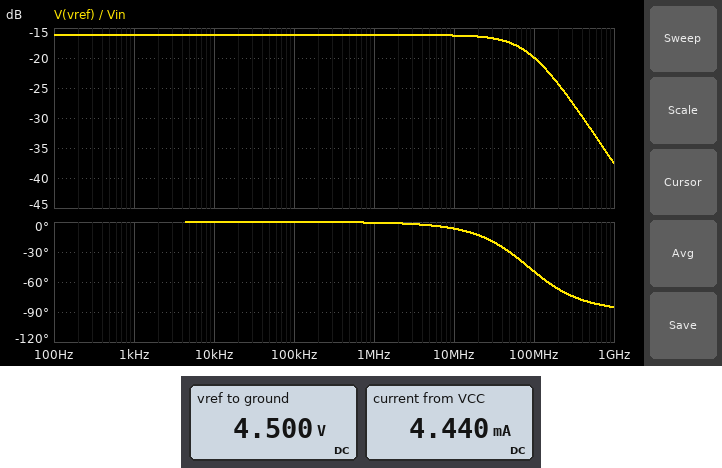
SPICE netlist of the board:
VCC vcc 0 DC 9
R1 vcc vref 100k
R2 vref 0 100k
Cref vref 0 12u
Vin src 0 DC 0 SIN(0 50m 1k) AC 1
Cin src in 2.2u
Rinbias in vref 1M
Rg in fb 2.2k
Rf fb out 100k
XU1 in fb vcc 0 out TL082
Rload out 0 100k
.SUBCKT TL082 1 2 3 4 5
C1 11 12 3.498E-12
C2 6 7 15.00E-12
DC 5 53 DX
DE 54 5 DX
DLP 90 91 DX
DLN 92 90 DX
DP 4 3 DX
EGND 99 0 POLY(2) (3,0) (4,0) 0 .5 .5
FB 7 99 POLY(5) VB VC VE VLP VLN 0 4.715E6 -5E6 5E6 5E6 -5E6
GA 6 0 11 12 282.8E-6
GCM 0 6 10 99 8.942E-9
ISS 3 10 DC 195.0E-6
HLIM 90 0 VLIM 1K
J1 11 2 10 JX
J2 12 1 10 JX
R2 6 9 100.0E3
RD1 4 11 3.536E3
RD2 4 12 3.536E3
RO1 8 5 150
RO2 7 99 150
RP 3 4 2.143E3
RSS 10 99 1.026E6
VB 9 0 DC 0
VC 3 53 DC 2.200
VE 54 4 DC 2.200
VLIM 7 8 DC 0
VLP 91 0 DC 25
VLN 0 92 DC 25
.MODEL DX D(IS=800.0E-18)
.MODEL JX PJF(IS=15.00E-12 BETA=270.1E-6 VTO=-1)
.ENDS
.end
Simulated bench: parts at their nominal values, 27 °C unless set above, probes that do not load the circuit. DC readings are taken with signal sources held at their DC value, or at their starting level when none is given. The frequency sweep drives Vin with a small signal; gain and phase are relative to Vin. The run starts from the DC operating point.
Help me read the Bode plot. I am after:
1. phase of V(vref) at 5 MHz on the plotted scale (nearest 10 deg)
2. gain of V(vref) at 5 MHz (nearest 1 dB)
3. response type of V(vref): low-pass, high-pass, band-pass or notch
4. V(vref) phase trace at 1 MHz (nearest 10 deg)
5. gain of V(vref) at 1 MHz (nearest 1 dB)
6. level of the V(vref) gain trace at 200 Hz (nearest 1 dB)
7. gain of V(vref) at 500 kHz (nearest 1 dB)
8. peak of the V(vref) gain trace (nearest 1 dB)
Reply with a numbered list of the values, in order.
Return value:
1. 0 deg
2. -16 dB
3. low-pass
4. 0 deg
5. -16 dB
6. -16 dB
7. -16 dB
8. -16 dB
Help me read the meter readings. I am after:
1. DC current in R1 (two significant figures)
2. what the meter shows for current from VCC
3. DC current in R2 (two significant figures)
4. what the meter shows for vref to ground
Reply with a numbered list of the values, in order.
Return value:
1. 45 µA
2. 4.440 mA
3. 45 µA
4. 4.500 V
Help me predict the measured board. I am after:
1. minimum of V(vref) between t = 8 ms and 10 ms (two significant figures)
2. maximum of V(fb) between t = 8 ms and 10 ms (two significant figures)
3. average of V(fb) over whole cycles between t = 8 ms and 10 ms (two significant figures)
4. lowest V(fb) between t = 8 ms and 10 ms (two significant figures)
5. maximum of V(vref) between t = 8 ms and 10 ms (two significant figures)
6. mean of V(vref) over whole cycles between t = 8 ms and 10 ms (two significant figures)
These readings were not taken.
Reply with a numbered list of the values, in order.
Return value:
1. 4.5 V
2. 4.5 V
3. 4.5 V
4. 4.5 V
5. 4.5 V
6. 4.5 V
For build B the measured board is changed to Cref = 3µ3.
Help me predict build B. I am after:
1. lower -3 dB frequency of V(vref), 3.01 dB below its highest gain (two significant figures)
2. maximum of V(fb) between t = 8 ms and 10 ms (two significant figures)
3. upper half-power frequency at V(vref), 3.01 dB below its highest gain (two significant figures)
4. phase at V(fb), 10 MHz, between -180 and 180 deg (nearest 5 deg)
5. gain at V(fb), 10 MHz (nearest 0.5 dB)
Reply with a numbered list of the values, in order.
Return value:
1. 580 mHz
2. 4.5 V
3. 120 MHz
4. 5 deg
5. -8.0 dB
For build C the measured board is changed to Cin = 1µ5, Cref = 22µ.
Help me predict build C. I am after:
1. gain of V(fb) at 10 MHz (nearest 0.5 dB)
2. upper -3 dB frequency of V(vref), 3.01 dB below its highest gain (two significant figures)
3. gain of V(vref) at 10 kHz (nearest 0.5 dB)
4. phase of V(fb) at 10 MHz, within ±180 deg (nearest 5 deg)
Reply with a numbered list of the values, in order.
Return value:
1. -19.5 dB
2. 110 MHz
3. -24.0 dB
4. 50 deg
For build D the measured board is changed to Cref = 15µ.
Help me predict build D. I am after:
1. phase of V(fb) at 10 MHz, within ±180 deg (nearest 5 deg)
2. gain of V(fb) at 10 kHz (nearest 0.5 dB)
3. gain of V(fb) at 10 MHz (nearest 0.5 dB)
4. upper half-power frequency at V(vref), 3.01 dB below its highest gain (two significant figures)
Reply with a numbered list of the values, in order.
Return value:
1. 35 deg
2. -18.0 dB
3. -15.5 dB
4. 83 MHz
